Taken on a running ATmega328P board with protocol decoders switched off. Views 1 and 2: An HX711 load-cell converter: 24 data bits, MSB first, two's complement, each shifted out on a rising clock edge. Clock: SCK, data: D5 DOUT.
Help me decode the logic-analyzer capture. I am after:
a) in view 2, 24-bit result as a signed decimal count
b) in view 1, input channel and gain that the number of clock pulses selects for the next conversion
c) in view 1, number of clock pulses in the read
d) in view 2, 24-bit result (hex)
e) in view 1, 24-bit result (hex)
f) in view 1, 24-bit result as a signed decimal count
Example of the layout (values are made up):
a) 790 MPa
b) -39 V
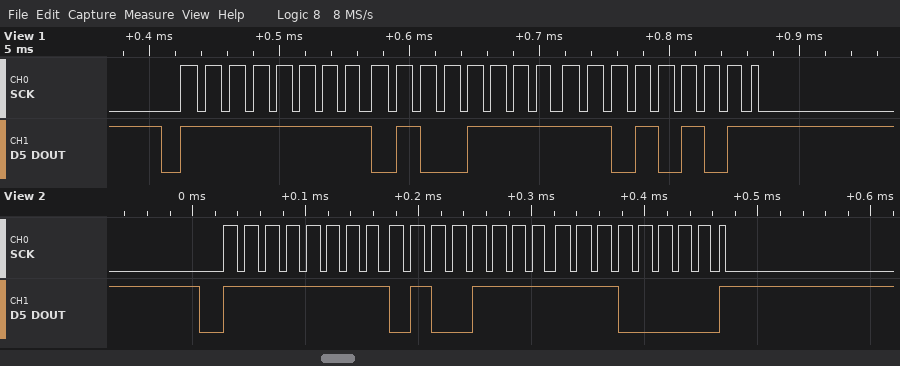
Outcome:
a) -45088
b) channel A, gain 128
c) 25
d) 0xFF4FE0
e) 0xFF4FD5
f) -45099
